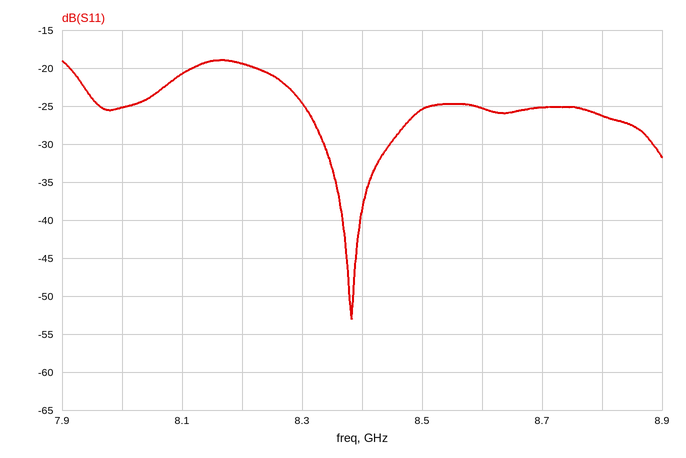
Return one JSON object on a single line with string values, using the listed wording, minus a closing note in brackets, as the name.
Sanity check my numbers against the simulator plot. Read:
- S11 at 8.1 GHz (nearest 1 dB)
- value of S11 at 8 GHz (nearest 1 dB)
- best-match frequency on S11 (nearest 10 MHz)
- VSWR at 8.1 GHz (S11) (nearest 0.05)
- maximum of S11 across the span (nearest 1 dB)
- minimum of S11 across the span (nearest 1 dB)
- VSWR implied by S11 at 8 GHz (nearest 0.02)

{"S11 at 8.1 GHz": "-21 dB", "value of S11 at 8 GHz": "-25 dB", "best-match frequency on S11": "8.38 GHz", "VSWR at 8.1 GHz (S11)": "1.20", "maximum of S11 across the span": "-19 dB", "minimum of S11 across the span": "-53 dB", "VSWR implied by S11 at 8 GHz": "1.12"}
